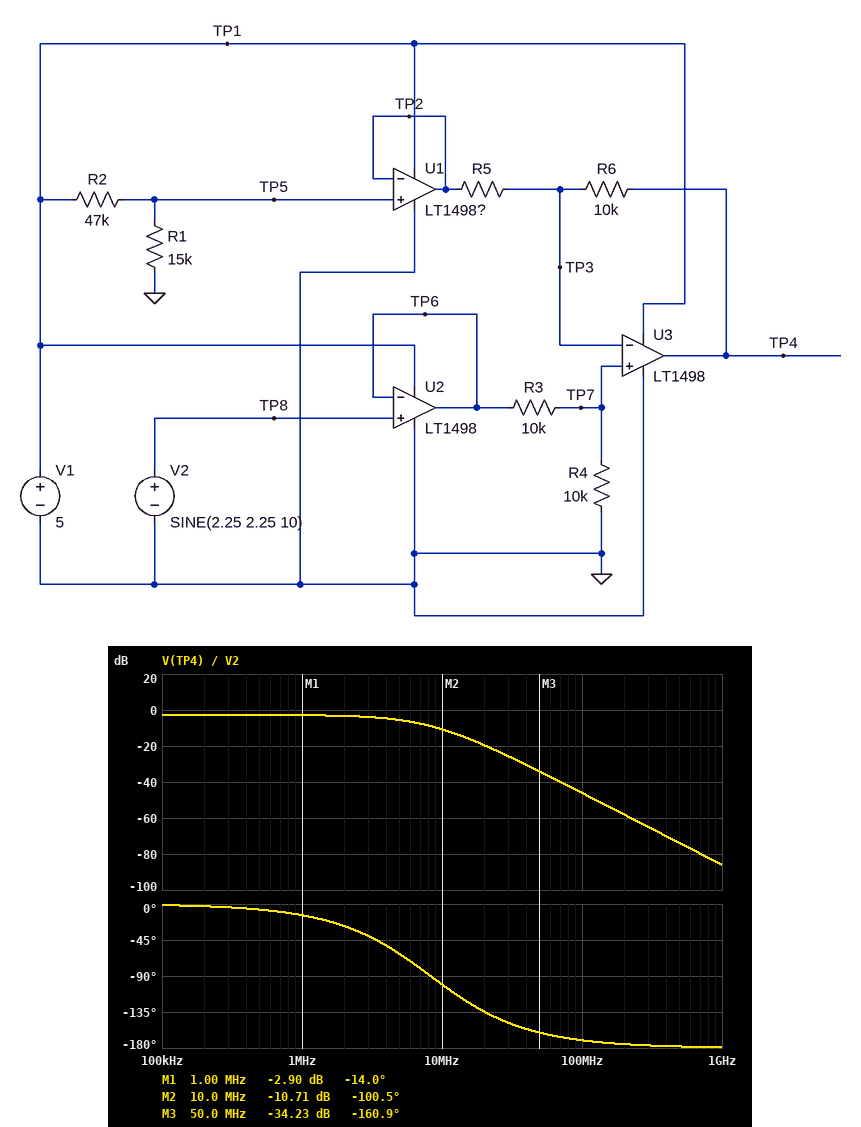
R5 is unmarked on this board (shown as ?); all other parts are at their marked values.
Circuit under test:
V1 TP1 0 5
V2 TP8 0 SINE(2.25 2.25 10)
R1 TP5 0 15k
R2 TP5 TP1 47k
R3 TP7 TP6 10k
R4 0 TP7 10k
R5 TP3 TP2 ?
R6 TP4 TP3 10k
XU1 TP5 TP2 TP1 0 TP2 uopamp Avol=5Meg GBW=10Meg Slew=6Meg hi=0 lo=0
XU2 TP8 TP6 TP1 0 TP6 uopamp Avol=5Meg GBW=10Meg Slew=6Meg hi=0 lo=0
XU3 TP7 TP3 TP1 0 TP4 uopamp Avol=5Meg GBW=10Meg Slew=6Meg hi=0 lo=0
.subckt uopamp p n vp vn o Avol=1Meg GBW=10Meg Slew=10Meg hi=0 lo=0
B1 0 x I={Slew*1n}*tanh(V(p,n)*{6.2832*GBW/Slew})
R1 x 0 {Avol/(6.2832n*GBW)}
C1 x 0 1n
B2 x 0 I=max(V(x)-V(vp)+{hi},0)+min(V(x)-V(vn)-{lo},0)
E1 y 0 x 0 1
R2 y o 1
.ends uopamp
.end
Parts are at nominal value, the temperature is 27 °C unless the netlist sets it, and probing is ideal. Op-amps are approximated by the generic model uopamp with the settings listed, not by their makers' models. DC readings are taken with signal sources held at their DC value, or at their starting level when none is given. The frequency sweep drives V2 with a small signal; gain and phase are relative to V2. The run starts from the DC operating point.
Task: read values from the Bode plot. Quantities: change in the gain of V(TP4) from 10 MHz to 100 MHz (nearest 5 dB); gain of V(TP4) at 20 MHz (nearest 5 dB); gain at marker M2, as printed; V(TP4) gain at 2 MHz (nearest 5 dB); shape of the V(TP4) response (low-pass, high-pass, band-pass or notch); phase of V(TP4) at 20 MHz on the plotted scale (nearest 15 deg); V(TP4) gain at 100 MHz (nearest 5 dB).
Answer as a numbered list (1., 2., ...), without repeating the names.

1. -35 dB
2. -20 dB
3. -10.71 dB
4. -5 dB
5. low-pass
6. -135 deg
7. -45 dB
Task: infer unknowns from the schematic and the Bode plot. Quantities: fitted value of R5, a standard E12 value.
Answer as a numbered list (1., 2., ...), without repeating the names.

1. 22 kΩ
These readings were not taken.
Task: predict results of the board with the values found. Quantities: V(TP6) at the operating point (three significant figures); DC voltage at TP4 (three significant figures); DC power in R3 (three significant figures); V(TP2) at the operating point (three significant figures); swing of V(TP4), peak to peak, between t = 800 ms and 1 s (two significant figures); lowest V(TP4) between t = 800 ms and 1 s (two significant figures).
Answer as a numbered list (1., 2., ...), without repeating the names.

1. 2.25 V
2. 1.09 V
3. 127 µW
4. 1.21 V
5. 2.7 V
6. -6.0 mV
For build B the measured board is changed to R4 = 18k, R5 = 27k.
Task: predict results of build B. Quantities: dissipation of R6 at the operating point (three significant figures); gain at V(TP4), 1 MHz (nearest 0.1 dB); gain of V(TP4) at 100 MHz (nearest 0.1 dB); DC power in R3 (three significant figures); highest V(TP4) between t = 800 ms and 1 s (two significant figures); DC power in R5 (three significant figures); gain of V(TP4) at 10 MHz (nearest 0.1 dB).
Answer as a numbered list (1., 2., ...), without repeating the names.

1. 769 nW
2. -1.2 dB
3. -43.9 dB
4. 64.6 µW
5. 3.5 V
6. 2.08 µW
7. -8.7 dB
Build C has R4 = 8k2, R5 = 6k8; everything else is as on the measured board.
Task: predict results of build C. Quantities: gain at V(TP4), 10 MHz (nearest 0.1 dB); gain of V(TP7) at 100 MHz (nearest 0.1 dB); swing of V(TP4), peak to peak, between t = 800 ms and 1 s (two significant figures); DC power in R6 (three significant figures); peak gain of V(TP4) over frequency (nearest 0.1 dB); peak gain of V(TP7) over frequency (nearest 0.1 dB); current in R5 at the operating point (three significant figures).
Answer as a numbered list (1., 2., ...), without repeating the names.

1. -10.6 dB
2. -27.0 dB
3. 3.2 V
4. 8.30 µW
5. 0.9 dB
6. -6.9 dB
7. 28.8 µA
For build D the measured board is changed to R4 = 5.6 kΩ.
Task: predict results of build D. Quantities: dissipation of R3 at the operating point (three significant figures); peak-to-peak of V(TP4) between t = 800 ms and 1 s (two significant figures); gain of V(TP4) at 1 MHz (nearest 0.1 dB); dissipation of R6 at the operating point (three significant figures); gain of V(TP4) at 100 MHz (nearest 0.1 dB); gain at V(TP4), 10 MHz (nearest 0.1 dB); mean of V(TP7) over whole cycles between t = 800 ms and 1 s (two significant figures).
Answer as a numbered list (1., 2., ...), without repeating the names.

1. 208 µW
2. 1.8 V
3. -5.8 dB
4. 3.34 µW
5. -49.0 dB
6. -13.6 dB
7. 810 mV
